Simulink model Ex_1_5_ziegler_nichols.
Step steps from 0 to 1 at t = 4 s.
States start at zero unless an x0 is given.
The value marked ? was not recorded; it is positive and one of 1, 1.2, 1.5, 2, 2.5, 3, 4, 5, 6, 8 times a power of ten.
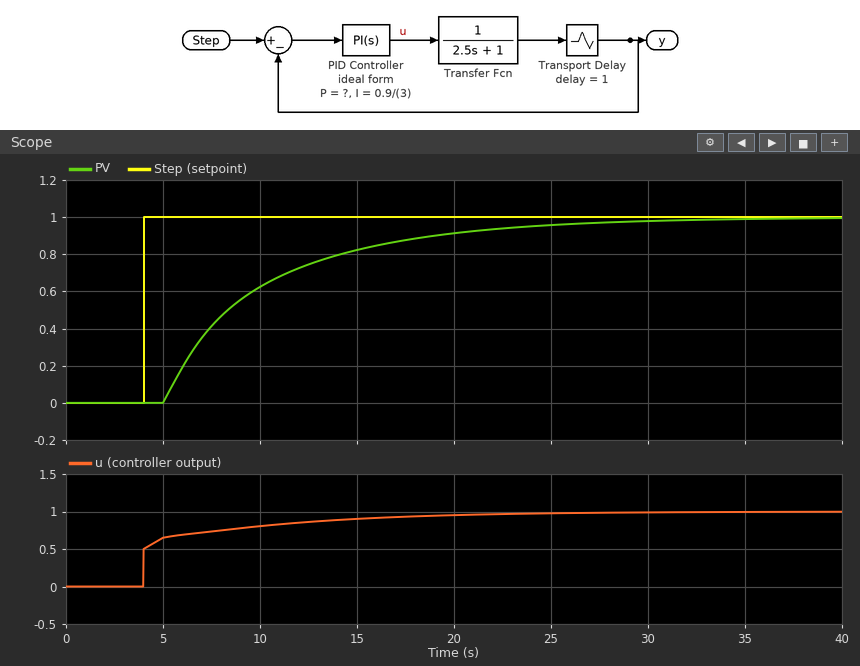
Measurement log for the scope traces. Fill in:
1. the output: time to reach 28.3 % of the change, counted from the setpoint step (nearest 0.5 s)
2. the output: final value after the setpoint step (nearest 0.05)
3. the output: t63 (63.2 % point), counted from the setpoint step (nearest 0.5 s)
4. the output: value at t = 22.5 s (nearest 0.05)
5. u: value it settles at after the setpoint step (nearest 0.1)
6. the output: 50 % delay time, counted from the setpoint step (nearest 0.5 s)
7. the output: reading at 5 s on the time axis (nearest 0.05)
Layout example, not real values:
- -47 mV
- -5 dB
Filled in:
- 2.5 s
- 1.00
- 6.0 s
- 0.95
- 1.0
- 4.5 s
- 0.00
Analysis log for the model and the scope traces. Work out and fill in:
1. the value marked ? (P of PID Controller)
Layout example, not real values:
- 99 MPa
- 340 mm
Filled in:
- 0.5
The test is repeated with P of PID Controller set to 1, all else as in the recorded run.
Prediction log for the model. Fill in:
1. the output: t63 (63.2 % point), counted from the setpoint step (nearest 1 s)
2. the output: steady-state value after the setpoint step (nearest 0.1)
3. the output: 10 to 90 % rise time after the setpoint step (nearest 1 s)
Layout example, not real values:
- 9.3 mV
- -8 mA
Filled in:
- 3 s
- 1.0
- 5 s
